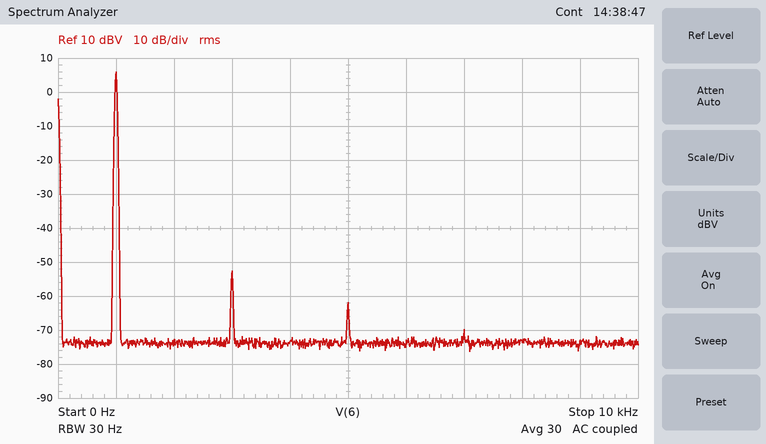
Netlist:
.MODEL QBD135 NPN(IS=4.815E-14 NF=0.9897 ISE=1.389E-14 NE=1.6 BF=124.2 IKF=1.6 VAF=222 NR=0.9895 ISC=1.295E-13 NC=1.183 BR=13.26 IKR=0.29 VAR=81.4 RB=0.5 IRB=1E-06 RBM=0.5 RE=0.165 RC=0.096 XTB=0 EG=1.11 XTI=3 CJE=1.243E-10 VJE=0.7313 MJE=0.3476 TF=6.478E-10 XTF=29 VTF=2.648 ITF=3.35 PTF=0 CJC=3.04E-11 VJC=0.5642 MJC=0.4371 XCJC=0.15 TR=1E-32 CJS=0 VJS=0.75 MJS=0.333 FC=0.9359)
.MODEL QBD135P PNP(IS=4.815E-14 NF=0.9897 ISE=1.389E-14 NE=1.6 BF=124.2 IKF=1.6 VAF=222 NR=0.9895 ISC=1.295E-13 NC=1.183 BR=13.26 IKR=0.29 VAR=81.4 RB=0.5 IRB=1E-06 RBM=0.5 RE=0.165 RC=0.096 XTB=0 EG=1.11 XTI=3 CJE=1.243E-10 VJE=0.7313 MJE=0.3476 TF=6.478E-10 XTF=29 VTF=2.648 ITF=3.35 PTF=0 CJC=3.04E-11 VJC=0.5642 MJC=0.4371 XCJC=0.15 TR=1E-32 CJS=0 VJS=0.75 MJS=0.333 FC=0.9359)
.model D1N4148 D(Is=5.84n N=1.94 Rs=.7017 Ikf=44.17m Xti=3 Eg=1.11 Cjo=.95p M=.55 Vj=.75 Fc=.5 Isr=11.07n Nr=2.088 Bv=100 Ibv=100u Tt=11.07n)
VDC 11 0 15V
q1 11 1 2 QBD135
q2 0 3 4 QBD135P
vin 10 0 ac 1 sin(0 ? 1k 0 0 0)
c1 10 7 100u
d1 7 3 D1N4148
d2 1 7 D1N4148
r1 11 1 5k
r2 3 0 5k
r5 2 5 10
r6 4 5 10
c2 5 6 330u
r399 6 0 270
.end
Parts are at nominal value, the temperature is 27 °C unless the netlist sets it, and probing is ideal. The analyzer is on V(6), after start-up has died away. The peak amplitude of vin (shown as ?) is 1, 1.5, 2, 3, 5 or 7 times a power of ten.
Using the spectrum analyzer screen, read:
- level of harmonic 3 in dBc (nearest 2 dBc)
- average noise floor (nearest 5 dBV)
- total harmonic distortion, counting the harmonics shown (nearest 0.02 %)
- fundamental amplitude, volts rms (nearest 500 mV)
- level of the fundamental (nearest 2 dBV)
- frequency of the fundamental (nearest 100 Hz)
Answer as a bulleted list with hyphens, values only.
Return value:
- -58 dBc
- -75 dBV
- 0.12 %
- 2.0 V
- 6 dBV
- 1.0 kHz
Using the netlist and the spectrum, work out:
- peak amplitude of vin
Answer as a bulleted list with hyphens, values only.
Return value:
- 3 V
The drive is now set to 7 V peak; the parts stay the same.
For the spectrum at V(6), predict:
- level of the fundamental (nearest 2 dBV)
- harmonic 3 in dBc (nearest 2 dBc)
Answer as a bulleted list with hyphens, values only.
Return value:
- 12 dBV
- -28 dBc
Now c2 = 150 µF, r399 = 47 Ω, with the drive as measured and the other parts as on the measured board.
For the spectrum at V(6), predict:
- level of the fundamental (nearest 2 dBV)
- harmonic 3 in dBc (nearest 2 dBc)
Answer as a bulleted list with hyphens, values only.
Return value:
- 4 dBV
- -46 dBc
